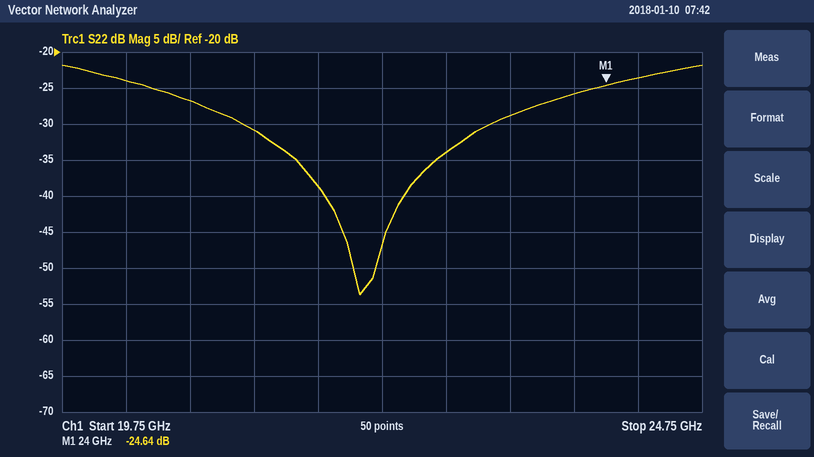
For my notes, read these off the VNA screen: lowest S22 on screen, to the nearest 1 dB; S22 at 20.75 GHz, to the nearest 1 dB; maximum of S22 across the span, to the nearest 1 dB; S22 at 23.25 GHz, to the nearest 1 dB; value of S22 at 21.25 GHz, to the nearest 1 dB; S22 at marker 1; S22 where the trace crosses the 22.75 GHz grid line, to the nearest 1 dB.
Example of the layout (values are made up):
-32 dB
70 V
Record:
-54 dB
-27 dB
-22 dB
-29 dB
-31 dB
-24.64 dB
-34 dB
